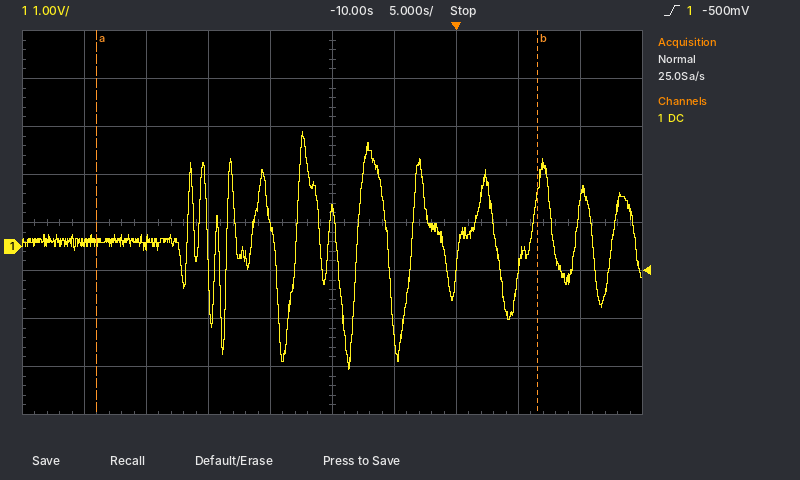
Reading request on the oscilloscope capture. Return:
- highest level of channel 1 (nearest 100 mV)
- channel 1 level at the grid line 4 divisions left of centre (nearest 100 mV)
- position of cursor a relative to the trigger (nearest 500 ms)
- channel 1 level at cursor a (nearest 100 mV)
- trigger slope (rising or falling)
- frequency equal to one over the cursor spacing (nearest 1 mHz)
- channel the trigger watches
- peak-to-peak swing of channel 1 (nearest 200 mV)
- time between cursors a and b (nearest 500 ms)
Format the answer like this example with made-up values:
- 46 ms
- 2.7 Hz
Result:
- 2.4 V
- 100 mV
- -29.0 s
- 100 mV
- rising
- 28 mHz
- channel 1
- 5.0 V
- 35.5 s
